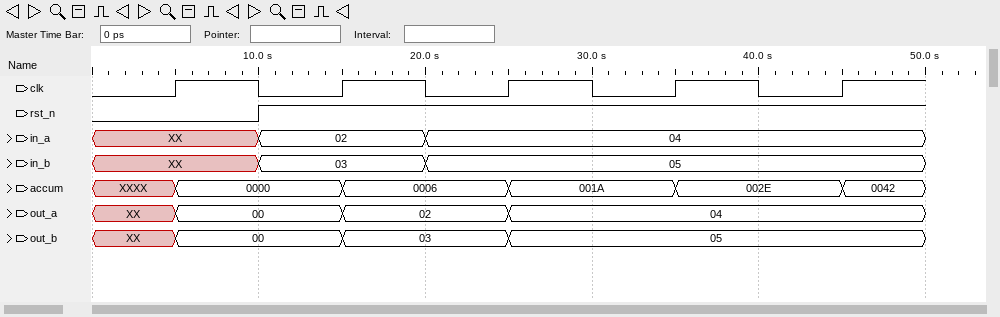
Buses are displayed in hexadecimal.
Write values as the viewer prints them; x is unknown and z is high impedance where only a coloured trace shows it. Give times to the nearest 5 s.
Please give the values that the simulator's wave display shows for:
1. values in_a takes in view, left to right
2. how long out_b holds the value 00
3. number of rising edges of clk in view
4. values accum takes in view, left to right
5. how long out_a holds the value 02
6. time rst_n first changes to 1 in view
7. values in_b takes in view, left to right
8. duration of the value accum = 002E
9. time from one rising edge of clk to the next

XX, 02, 04
10 s
5
XXXX, 0000, 0006, 001A, 002E, 0042
10 s
10 s
XX, 03, 05
10 s
10 s
